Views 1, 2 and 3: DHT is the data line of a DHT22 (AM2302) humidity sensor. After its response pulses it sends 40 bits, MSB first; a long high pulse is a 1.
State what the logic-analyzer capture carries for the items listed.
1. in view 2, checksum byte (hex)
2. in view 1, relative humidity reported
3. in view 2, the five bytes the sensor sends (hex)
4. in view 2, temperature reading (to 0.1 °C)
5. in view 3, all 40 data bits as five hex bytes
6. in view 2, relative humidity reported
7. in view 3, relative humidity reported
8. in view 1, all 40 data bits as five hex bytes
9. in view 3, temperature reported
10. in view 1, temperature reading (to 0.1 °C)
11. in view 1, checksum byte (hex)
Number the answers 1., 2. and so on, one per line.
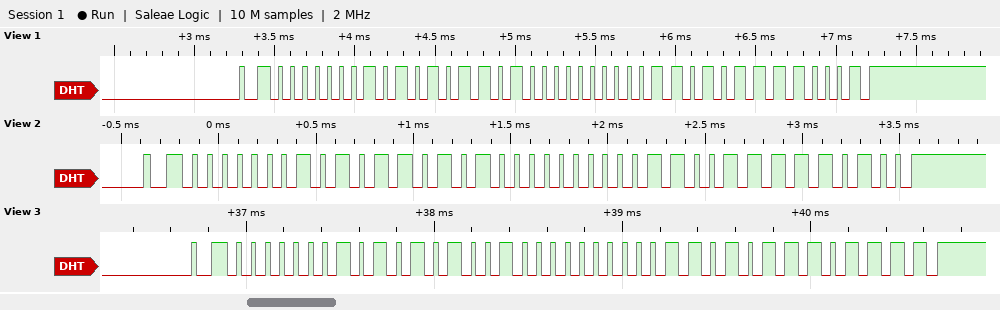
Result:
1. 0xF4
2. 34.2 %
3. 01 5A 80 19 F4
4. -2.5 °C
5. 01 54 80 1A EF
6. 34.6 %
7. 34.0 %
8. 01 56 80 1A F1
9. -2.6 °C
10. -2.6 °C
11. 0xF1
